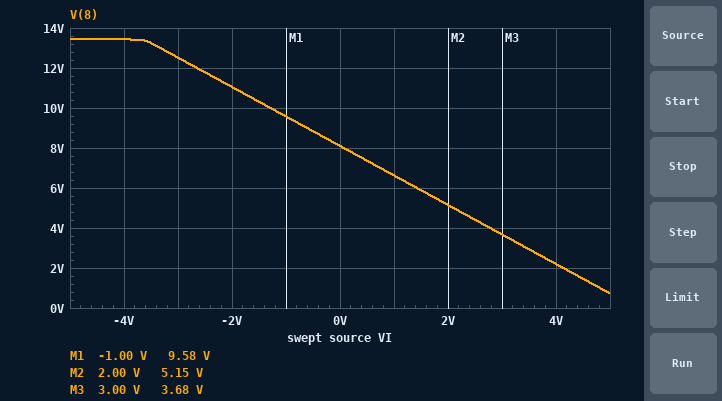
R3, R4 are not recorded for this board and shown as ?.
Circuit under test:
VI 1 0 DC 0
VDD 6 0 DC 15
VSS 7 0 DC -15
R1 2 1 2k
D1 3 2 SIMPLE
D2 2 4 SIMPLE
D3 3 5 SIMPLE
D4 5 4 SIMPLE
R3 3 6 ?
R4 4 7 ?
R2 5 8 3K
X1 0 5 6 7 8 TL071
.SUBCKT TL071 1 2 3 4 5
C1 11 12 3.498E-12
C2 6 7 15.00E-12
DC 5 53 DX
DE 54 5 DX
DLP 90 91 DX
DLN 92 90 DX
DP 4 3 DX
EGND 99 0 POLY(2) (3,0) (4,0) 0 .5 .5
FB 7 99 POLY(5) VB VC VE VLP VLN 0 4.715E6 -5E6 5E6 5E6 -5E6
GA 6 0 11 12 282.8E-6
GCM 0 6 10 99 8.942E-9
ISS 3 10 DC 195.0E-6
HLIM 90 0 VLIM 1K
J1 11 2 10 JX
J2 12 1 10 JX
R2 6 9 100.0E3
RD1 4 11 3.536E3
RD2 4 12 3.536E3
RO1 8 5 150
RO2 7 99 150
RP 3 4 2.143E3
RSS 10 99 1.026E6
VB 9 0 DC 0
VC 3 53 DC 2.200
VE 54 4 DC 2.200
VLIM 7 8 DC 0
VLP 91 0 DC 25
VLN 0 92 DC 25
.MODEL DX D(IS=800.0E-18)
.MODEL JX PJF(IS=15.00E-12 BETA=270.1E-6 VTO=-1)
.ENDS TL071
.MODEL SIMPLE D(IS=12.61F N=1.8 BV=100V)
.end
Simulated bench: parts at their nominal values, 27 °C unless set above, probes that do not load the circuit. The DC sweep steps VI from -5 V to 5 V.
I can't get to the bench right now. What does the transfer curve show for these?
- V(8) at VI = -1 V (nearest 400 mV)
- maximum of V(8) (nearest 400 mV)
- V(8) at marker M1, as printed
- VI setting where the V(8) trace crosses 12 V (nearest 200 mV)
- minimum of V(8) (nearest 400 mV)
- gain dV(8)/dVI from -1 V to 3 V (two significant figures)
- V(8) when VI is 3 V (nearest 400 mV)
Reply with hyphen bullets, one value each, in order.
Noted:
- 9.6 V
- 13.6 V
- 9.58 V
- -2.6 V
- 800 mV
- -1.5 V/V
- 3.6 V
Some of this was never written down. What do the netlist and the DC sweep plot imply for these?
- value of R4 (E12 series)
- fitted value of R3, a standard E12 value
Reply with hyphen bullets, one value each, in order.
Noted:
- 2.2 kΩ
- 3.9 kΩ
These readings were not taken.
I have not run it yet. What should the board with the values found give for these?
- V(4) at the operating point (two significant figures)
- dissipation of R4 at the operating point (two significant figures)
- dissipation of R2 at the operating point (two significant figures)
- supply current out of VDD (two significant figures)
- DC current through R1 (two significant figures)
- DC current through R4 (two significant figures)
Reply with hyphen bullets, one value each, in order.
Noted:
- -1.2 V
- 86 mW
- 22 mW
- 18 mA
- 13 µA
- 6.3 mA
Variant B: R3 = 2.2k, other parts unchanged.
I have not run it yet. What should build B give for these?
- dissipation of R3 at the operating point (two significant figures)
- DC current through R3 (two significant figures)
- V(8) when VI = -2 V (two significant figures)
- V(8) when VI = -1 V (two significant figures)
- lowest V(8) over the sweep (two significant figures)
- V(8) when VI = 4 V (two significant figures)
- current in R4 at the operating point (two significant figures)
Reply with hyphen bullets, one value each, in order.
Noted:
- 86 mW
- 6.3 mA
- 3.0 V
- 1.5 V
- -7.4 V
- -5.9 V
- 6.3 mA
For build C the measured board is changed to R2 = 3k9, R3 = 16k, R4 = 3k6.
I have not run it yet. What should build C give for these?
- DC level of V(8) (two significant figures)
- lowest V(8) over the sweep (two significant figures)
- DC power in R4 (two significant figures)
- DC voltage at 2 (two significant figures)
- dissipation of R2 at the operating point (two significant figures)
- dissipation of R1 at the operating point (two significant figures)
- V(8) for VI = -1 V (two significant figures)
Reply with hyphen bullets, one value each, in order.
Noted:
- 11 V
- 1.9 V
- 53 mW
- -67 mV
- 33 mW
- 2.2 µW
- 13 V
